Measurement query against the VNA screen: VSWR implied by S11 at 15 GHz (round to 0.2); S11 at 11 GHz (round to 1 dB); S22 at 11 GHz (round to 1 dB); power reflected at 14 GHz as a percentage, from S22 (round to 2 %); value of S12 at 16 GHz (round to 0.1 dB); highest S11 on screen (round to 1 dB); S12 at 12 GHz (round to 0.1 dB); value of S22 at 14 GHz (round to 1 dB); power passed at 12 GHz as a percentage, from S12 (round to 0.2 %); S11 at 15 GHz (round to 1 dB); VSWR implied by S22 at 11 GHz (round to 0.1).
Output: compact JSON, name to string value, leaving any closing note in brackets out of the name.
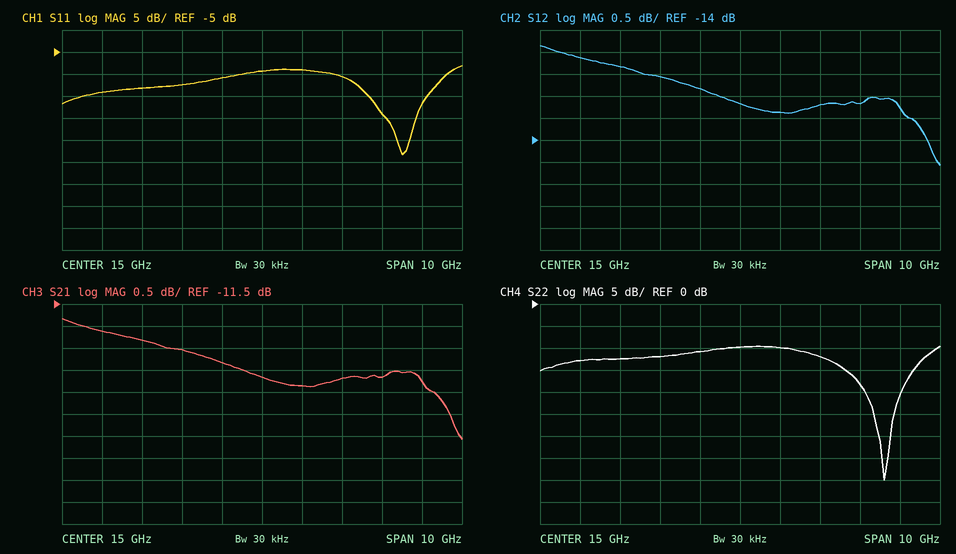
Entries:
{"VSWR implied by S11 at 15 GHz": "2.0", "S11 at 11 GHz": "-14 dB", "S22 at 11 GHz": "-13 dB", "power reflected at 14 GHz as a percentage, from S22": "8 %", "value of S12 at 16 GHz": "-13.4 dB", "highest S11 on screen": "-8 dB", "S12 at 12 GHz": "-12.3 dB", "value of S22 at 14 GHz": "-11 dB", "power passed at 12 GHz as a percentage, from S12": "5.8 %", "S11 at 15 GHz": "-9 dB", "VSWR implied by S22 at 11 GHz": "1.6"}
